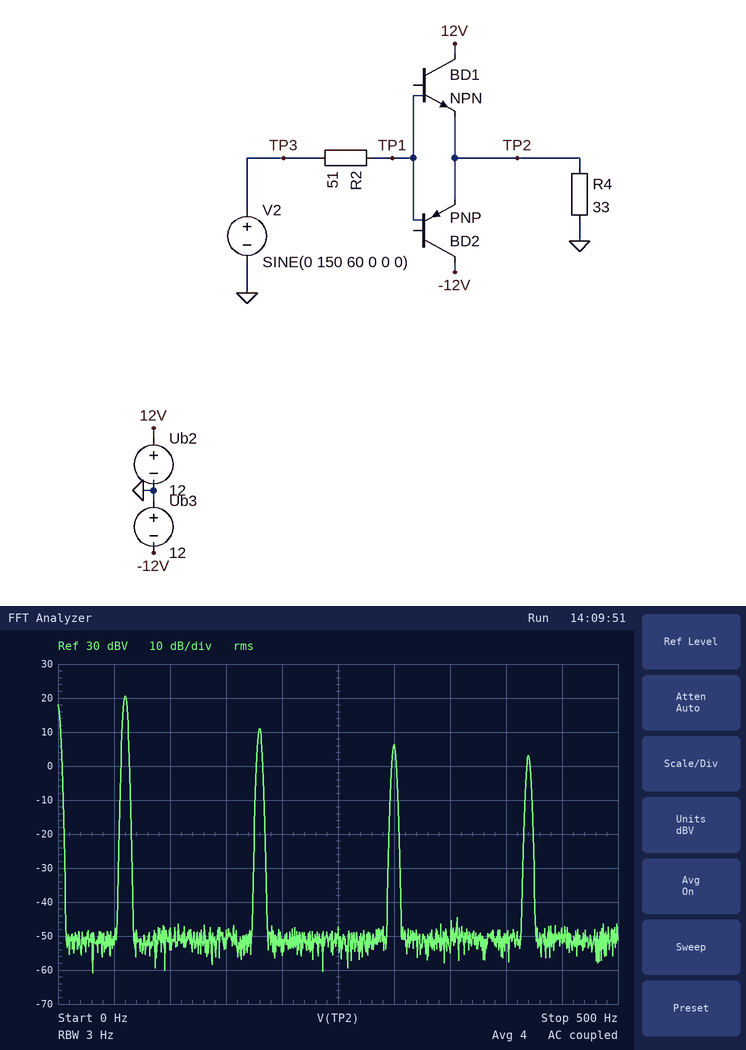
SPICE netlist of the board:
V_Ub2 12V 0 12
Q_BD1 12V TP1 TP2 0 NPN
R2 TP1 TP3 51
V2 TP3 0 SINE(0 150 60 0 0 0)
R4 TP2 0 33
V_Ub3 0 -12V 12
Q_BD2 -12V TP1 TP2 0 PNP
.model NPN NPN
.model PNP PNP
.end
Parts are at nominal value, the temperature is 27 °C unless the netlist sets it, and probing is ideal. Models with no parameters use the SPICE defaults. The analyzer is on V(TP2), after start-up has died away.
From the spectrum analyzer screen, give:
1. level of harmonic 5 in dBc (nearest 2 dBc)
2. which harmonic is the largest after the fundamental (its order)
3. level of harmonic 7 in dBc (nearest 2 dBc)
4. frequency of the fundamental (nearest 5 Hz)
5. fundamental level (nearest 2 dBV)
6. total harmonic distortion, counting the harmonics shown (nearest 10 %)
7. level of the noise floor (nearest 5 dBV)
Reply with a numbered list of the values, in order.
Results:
1. -14 dBc
2. 3
3. -18 dBc
4. 60 Hz
5. 20 dBV
6. 40 %
7. -50 dBV
